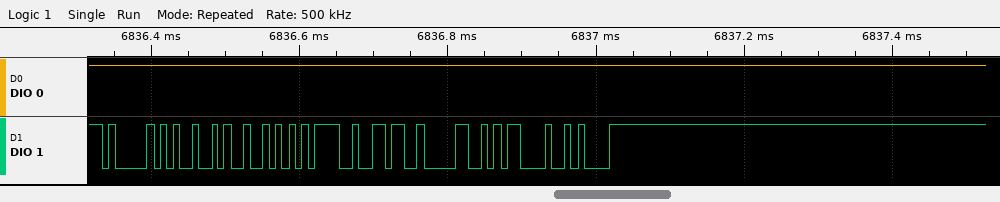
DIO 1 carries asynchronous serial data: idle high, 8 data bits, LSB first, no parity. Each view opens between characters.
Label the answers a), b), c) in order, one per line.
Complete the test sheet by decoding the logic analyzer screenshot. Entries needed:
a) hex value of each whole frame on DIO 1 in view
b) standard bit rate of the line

a) 41, 49, 52, 3D, 36, 30, 0D, 0A
b) 115200 baud
